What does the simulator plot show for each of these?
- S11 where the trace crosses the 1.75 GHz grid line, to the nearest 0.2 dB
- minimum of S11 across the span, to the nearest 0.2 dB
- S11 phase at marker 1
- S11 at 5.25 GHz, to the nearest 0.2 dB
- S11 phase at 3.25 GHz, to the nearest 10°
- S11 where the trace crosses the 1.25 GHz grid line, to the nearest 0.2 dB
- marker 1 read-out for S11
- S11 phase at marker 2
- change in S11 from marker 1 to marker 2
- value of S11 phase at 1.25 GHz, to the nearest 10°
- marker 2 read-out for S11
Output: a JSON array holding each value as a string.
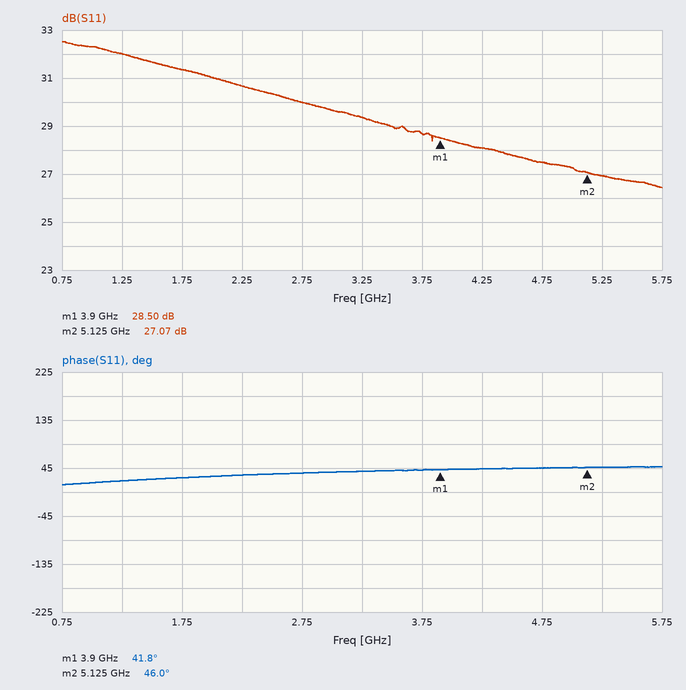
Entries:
["31.4 dB", "26.4 dB", "41.8°", "27.0 dB", "40°", "32.0 dB", "28.50 dB", "46.0°", "-1.43 dB", "20°", "27.07 dB"]
